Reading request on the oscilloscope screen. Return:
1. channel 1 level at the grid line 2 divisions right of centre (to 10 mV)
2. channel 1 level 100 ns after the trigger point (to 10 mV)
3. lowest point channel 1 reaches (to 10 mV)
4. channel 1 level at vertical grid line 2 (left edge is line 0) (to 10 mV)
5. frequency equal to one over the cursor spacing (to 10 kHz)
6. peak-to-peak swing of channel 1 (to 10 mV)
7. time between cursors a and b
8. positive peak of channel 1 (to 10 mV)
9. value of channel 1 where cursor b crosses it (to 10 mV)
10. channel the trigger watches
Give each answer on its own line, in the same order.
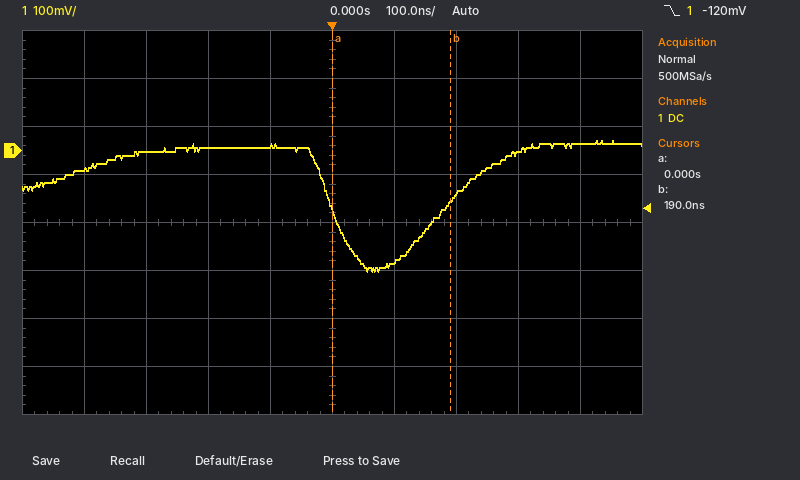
-90 mV
-230 mV
-250 mV
0 mV
5.26 MHz
270 mV
190 ns
20 mV
-110 mV
channel 1
